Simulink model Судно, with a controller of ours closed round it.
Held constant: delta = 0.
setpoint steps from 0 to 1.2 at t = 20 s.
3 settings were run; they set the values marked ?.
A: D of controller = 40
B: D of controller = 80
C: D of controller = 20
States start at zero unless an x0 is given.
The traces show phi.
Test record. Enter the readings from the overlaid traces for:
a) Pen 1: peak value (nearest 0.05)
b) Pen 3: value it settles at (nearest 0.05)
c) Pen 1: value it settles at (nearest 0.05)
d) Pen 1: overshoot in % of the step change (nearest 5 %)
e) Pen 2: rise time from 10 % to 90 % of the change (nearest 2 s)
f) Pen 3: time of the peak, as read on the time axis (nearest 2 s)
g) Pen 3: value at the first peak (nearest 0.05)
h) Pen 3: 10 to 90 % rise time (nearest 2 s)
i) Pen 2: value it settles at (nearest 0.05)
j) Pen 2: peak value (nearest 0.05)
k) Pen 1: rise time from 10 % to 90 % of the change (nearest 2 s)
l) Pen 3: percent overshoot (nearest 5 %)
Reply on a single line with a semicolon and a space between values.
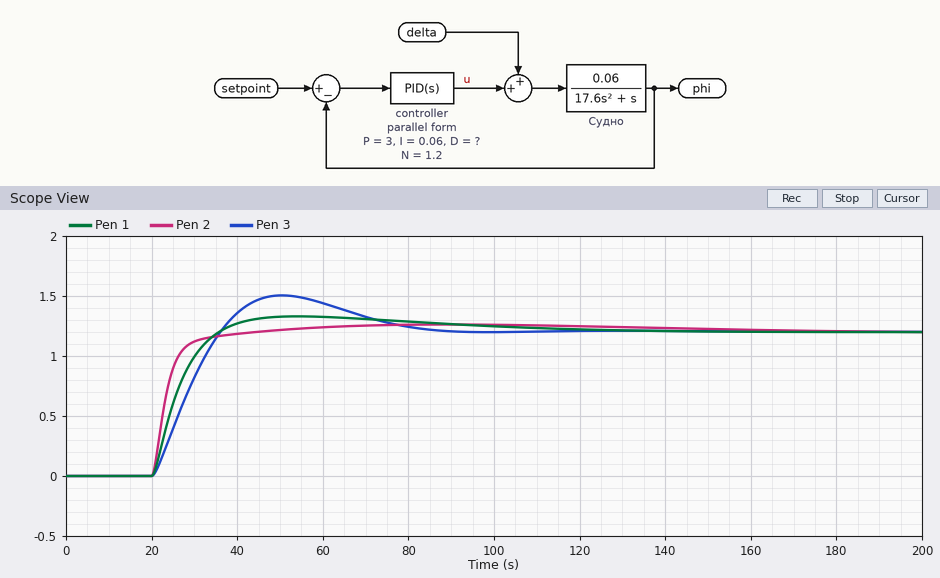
1.35; 1.20; 1.20; 10 %; 8 s; 50 s; 1.50; 12 s; 1.20; 1.25; 10 s; 25 %
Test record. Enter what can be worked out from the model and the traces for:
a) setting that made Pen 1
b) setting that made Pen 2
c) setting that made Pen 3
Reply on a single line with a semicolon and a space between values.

A; B; C
